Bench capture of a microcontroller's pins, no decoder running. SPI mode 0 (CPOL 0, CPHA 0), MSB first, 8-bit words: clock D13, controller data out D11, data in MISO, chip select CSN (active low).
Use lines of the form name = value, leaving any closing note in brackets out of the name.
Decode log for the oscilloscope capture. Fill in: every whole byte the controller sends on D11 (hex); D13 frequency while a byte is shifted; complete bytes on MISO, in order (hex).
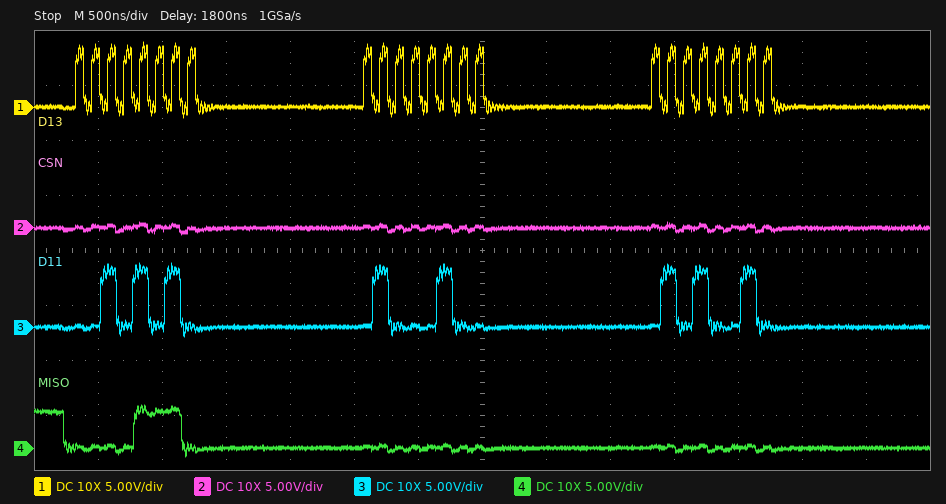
every whole byte the controller sends on D11 = 2A 44 52
D13 frequency while a byte is shifted = 8 MHz
complete bytes on MISO, in order = 0E 00 00
